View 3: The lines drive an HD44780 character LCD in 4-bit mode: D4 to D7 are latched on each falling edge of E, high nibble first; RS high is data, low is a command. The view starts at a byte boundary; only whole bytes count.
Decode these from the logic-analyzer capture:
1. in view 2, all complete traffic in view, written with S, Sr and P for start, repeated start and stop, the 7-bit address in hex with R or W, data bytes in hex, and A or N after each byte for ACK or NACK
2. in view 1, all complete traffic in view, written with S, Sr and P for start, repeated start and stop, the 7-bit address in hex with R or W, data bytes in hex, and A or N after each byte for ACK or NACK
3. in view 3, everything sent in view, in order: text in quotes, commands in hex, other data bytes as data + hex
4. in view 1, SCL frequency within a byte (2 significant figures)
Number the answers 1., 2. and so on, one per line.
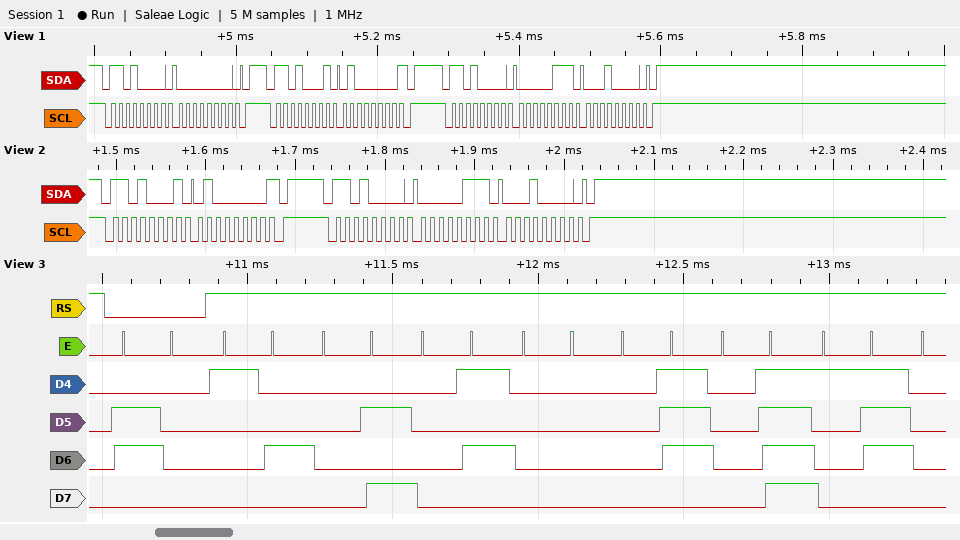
1. S 68R A 40 N P S 68W A 07 A 10 A P
2. S 68W A 00 A P S 68R A 40 N P S 68W A 07 A 10 A P
3. 0x60 data 14 0A 05 00 07 0F 17
4. 100 kHz
